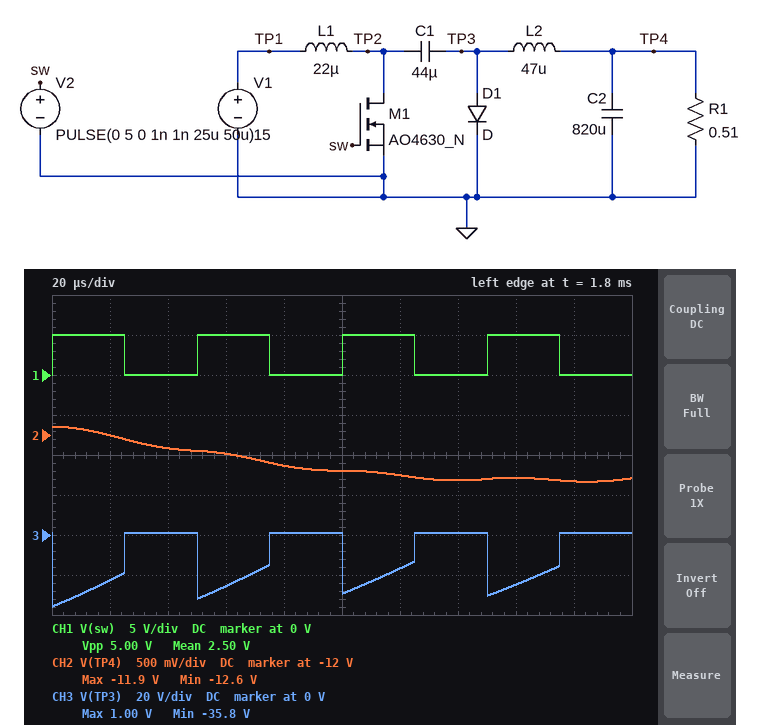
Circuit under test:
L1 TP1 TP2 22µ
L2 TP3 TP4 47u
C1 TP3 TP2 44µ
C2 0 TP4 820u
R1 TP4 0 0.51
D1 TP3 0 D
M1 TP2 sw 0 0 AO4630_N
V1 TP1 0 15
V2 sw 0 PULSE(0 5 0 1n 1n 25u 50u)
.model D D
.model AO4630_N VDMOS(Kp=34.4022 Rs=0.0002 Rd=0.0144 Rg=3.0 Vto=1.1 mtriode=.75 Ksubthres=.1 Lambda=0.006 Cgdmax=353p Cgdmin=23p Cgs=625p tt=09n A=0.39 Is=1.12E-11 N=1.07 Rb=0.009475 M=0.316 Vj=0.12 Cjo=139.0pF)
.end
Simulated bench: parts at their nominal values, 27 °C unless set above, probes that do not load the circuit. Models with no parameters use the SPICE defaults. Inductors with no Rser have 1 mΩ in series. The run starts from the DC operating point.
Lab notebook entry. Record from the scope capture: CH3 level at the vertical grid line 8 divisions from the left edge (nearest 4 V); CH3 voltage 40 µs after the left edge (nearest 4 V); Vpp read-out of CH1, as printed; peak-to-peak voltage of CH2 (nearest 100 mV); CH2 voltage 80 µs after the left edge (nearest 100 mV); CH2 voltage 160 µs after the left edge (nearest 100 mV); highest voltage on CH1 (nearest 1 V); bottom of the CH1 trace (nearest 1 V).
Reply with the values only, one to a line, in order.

-24 V
0 V
5.00 V
700 mV
-12.4 V
-12.5 V
5 V
0 V
